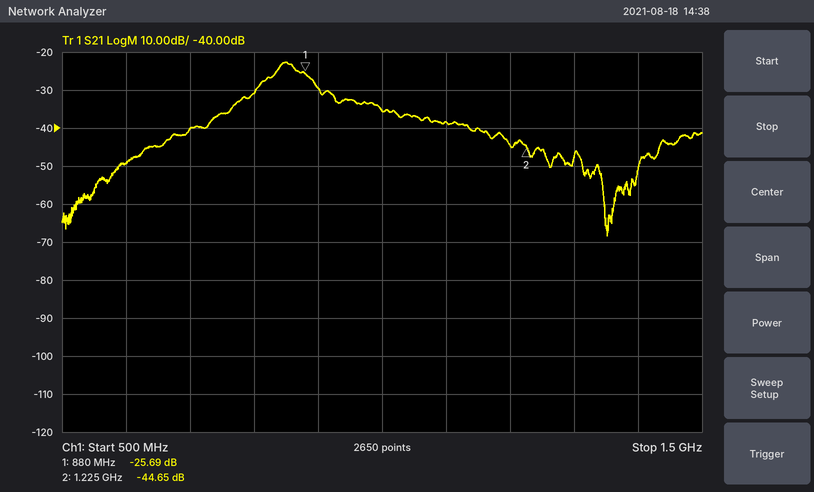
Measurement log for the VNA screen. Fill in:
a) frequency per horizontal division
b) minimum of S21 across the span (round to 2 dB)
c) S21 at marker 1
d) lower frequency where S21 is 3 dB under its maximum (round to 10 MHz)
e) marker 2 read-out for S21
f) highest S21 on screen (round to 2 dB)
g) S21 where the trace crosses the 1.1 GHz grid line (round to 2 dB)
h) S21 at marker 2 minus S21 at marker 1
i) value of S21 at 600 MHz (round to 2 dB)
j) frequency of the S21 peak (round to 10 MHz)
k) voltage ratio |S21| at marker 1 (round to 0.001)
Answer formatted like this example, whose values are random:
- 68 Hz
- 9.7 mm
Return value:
- 100 MHz
- -68 dB
- -25.69 dB
- 830 MHz
- -44.65 dB
- -22 dB
- -38 dB
- -18.96 dB
- -50 dB
- 850 MHz
- 0.052
